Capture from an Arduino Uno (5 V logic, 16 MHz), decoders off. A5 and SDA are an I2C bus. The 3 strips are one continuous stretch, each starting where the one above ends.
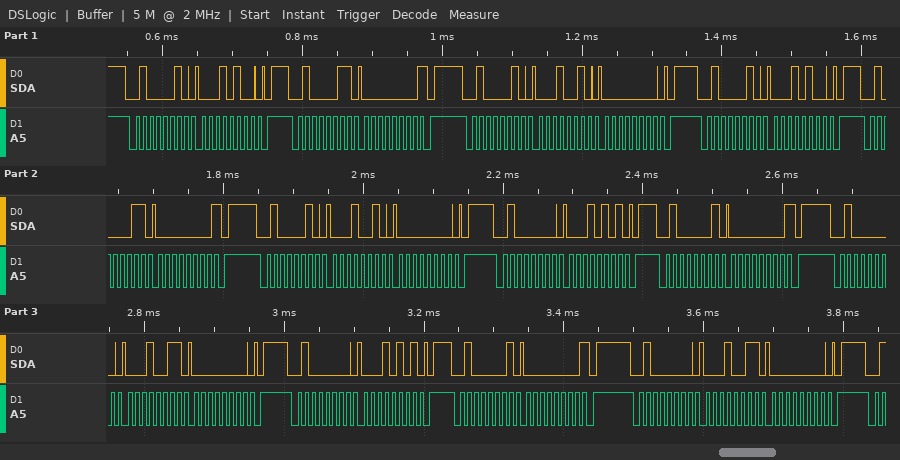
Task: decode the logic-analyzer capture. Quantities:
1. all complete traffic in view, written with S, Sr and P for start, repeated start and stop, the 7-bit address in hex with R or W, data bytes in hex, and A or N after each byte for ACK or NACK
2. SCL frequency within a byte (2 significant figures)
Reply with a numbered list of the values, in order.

1. S 21W A 14 A P S 21R A 00 N P S 21W A 12 A 00 A P S 21W A 14 A P S 21R A 00 N P S 21W A 12 A 00 A P S 20W A 15 A P S 20R A 00 N P S 20W A 13 A 00 A P S 20W A 15 A P S 20R A 00 N P S 20W A 13 A 00 A P
2. 100 kHz
